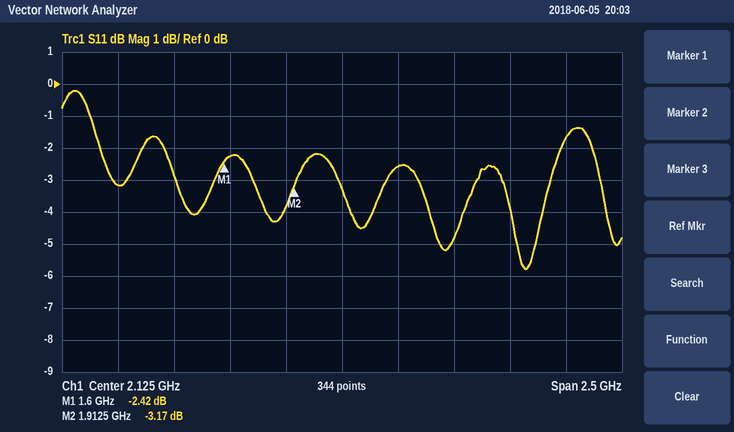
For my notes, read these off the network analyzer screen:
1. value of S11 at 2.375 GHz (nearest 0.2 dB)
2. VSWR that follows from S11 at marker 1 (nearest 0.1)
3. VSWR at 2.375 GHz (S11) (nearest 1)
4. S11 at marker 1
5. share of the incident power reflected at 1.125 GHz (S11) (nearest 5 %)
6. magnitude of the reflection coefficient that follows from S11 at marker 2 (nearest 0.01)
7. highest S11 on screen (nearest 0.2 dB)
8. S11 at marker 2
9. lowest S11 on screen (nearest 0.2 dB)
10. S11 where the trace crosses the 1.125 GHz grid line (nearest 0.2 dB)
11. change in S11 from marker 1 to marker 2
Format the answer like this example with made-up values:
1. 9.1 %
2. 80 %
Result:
1. -2.6 dB
2. 7.2
3. 7
4. -2.42 dB
5. 50 %
6. 0.69
7. -0.2 dB
8. -3.17 dB
9. -5.8 dB
10. -3.2 dB
11. -0.75 dB
